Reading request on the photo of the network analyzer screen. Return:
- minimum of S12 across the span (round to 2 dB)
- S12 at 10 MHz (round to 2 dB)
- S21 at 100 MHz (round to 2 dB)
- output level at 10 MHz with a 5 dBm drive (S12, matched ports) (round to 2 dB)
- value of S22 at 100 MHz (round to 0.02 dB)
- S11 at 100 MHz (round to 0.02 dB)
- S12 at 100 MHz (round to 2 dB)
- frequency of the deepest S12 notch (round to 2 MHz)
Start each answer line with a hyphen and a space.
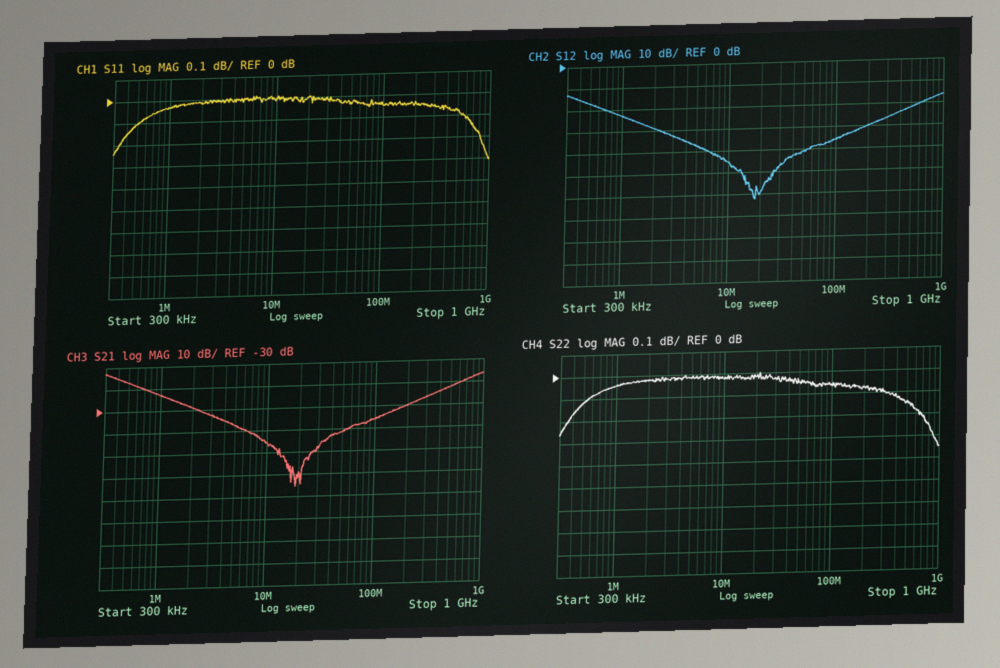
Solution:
- -62 dB
- -46 dB
- -36 dB
- -40 dBm
- -0.06 dB
- -0.04 dB
- -36 dB
- 18 MHz
